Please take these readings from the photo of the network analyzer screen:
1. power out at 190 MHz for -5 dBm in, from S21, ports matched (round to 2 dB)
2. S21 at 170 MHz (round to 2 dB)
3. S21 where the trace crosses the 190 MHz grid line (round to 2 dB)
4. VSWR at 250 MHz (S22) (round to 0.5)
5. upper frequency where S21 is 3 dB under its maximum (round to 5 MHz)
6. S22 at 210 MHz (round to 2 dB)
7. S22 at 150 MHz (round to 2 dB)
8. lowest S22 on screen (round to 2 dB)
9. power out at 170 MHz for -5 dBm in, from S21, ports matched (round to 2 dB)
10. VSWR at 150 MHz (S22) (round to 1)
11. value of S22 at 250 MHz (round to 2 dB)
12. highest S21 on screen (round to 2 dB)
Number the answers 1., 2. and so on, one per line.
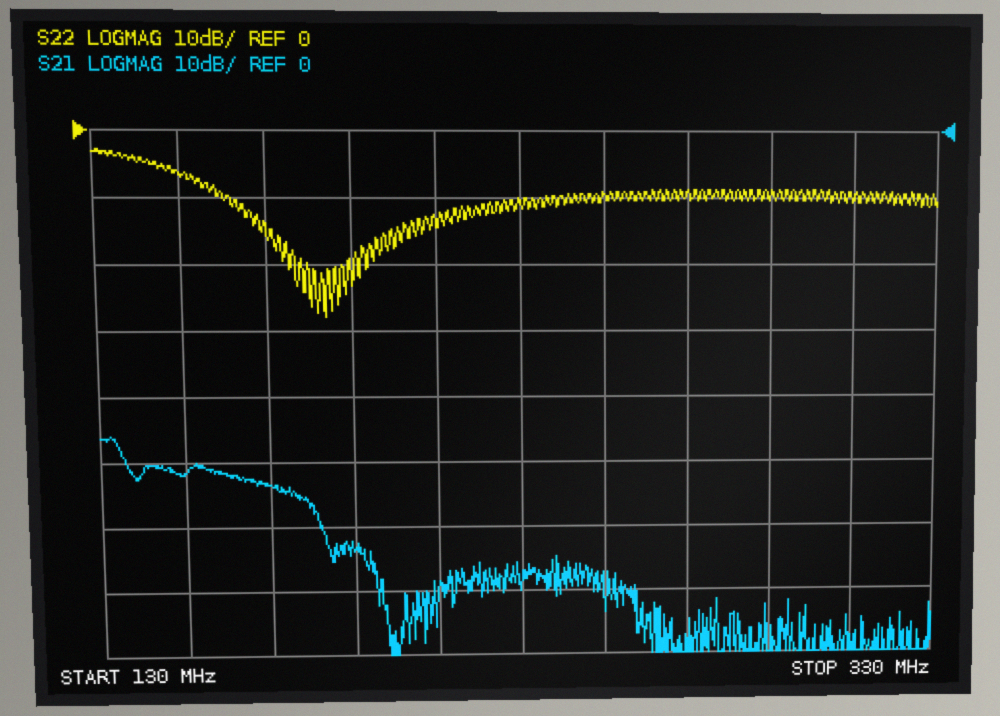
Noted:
1. -68 dBm
2. -54 dB
3. -64 dB
4. 2.0
5. 135 MHz
6. -14 dB
7. -6 dB
8. -28 dB
9. -58 dBm
10. 3
11. -10 dB
12. -46 dB
